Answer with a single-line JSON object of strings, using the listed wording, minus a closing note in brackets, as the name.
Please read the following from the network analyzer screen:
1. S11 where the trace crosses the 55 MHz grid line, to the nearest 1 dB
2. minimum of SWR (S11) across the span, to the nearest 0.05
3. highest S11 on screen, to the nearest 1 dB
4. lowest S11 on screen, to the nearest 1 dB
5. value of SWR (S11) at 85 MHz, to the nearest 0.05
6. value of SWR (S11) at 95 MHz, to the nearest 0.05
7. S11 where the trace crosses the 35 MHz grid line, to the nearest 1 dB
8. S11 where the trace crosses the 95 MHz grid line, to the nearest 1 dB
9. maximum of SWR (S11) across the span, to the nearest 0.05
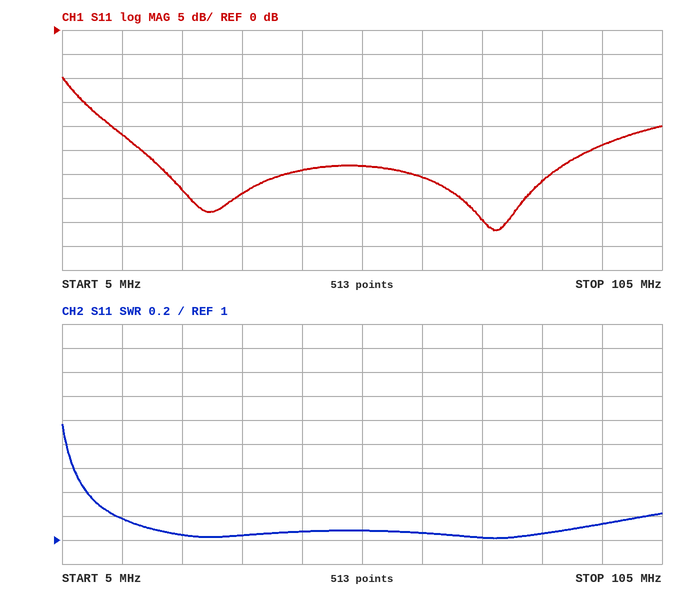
{"S11 where the trace crosses the 55 MHz grid line, to the nearest 1 dB": "-28 dB", "minimum of SWR (S11) across the span, to the nearest 0.05": "1.00", "highest S11 on screen, to the nearest 1 dB": "-10 dB", "lowest S11 on screen, to the nearest 1 dB": "-42 dB", "value of SWR (S11) at 85 MHz, to the nearest 0.05": "1.05", "value of SWR (S11) at 95 MHz, to the nearest 0.05": "1.15", "S11 where the trace crosses the 35 MHz grid line, to the nearest 1 dB": "-34 dB", "S11 where the trace crosses the 95 MHz grid line, to the nearest 1 dB": "-24 dB", "maximum of SWR (S11) across the span, to the nearest 0.05": "1.95"}
